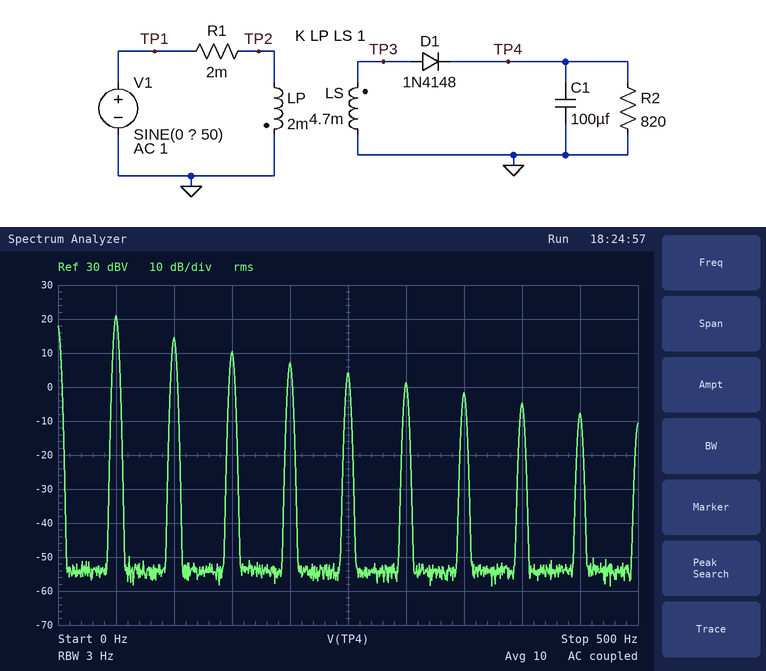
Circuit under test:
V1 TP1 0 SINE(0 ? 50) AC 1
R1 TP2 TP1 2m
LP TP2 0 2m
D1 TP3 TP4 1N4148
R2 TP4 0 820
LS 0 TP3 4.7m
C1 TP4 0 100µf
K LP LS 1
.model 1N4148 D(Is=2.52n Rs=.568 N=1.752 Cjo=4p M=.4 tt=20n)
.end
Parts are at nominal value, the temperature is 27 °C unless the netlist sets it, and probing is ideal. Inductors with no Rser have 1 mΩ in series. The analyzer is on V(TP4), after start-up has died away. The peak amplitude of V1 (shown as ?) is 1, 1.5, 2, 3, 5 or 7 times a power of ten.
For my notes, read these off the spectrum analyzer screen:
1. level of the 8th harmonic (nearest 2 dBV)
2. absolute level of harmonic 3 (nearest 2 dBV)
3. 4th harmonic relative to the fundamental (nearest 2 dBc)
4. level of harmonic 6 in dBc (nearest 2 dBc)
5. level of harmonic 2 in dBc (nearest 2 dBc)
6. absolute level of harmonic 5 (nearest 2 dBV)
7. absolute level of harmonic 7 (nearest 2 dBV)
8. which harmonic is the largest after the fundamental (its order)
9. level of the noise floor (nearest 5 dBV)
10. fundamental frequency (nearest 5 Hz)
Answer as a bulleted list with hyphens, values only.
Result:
- -4 dBV
- 10 dBV
- -14 dBc
- -20 dBc
- -6 dBc
- 4 dBV
- -2 dBV
- 2
- -55 dBV
- 50 Hz
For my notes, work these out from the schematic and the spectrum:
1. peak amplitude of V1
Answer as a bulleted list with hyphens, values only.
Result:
- 150 V
